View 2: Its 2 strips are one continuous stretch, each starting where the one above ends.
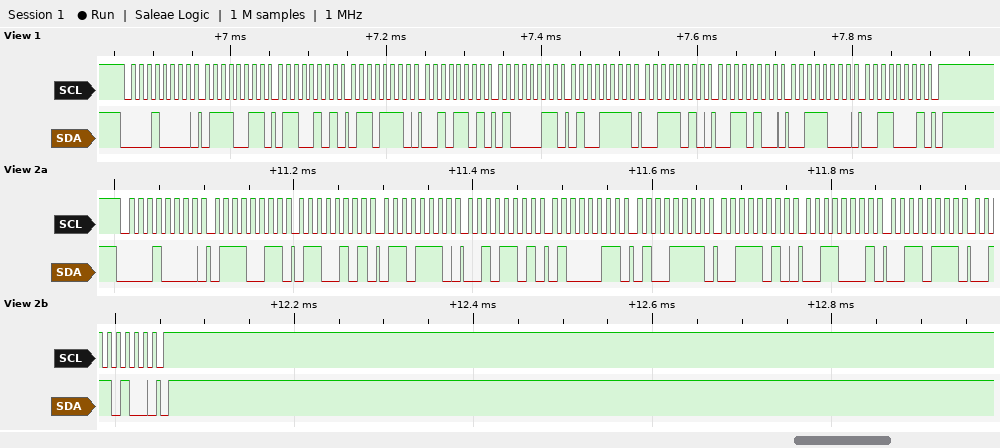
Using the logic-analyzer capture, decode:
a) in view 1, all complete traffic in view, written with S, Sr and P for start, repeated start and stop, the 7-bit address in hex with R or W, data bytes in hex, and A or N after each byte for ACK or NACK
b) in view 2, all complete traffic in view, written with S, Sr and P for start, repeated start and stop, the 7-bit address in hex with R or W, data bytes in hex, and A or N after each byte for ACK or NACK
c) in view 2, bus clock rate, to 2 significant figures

S 08W A 73 A 65 A 6E A 2D A 43 A 4F A 3A A 34 A 38 A 31 A P
S 08W A 73 A 65 A 6E A 2D A 43 A 4F A 3A A 31 A 37 A 34 A P
100 kHz
